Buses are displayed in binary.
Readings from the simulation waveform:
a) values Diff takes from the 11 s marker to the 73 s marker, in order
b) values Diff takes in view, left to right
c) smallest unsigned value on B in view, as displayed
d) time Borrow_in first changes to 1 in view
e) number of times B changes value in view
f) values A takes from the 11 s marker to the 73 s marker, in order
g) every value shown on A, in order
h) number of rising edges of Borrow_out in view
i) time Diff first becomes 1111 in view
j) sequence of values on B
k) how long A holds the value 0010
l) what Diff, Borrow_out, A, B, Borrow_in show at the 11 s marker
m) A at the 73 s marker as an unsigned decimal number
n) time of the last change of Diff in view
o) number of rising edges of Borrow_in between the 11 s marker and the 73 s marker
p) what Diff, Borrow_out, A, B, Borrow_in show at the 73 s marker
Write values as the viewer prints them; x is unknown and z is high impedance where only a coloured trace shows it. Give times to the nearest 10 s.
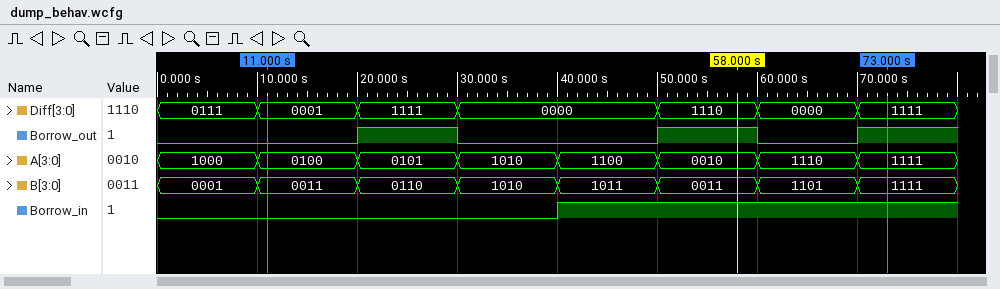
0001, 1111, 0000, 1110, 0000, 1111
0111, 0001, 1111, 0000, 1110, 0000, 1111
0001
40 s
7
0100, 0101, 1010, 1100, 0010, 1110, 1111
1000, 0100, 0101, 1010, 1100, 0010, 1110, 1111
3
20 s
0001, 0011, 0110, 1010, 1011, 0011, 1101, 1111
10 s
Diff=0001, Borrow_out=0, A=0100, B=0011, Borrow_in=0
15
70 s
1
Diff=1111, Borrow_out=1, A=1111, B=1111, Borrow_in=1
